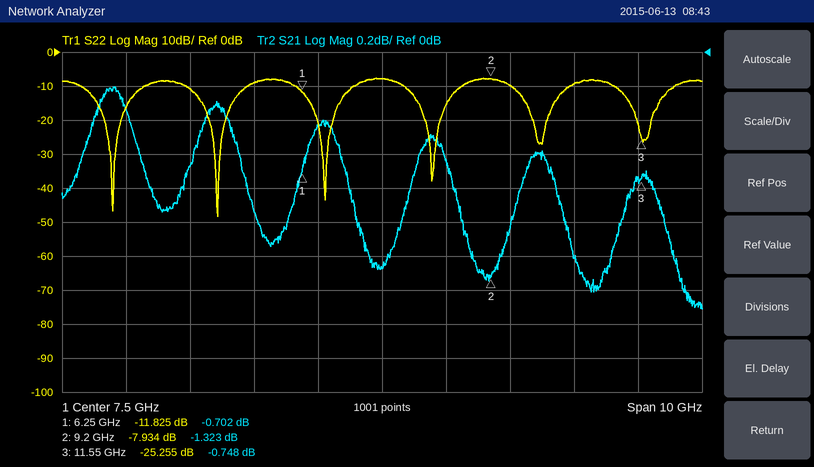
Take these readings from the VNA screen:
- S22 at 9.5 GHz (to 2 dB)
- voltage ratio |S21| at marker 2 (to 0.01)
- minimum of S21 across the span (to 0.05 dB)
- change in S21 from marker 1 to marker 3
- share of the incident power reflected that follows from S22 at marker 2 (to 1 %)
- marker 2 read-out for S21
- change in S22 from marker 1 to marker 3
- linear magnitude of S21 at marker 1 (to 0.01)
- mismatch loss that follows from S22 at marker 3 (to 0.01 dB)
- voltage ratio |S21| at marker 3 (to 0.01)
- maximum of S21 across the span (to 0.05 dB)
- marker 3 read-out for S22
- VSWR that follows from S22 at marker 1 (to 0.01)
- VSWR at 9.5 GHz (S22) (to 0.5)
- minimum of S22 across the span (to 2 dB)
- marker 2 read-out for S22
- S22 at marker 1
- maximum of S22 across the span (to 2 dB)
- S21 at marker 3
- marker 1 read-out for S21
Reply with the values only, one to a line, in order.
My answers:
-10 dB
0.86
-1.50 dB
-0.046 dB
16 %
-1.323 dB
-13.430 dB
0.92
0.01 dB
0.92
-0.20 dB
-25.255 dB
1.69
2.0
-48 dB
-7.934 dB
-11.825 dB
-8 dB
-0.748 dB
-0.702 dB
